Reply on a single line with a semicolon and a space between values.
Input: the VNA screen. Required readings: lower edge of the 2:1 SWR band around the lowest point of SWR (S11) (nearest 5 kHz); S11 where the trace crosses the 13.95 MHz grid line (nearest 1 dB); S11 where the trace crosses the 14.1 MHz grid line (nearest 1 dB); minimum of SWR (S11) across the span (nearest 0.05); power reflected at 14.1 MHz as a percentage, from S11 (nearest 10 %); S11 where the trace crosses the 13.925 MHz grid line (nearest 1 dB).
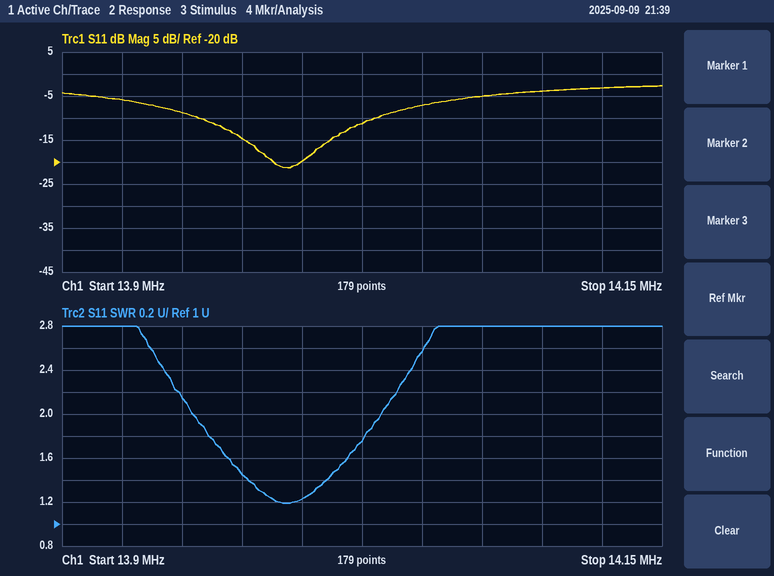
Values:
13.955 MHz; -9 dB; -4 dB; 1.20; 40 %; -6 dB
